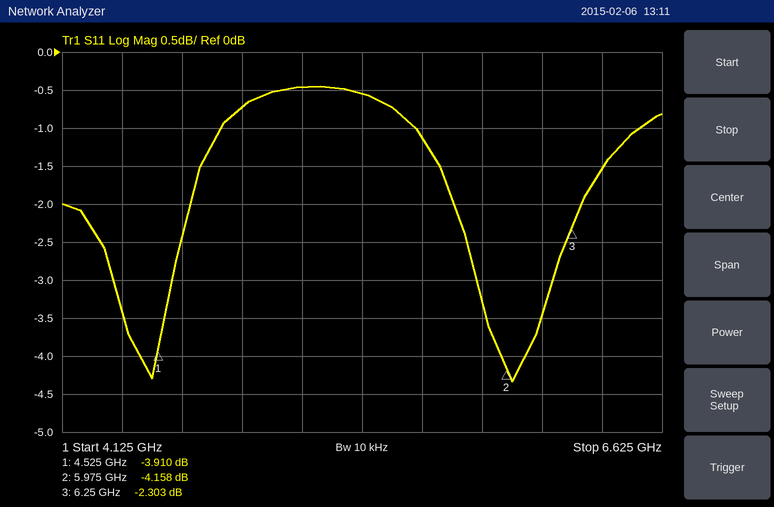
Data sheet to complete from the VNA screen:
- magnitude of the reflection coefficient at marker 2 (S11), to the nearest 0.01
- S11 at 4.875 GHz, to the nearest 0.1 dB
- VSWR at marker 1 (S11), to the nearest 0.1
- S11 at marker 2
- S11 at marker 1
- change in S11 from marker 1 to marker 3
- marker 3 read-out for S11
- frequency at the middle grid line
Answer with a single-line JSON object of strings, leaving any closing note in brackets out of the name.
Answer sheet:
{"magnitude of the reflection coefficient at marker 2 (S11), to the nearest 0.01": "0.62", "S11 at 4.875 GHz, to the nearest 0.1 dB": "-0.7 dB", "VSWR at marker 1 (S11), to the nearest 0.1": "4.5", "S11 at marker 2": "-4.158 dB", "S11 at marker 1": "-3.910 dB", "change in S11 from marker 1 to marker 3": "1.607 dB", "marker 3 read-out for S11": "-2.303 dB", "frequency at the middle grid line": "5.375 GHz"}
